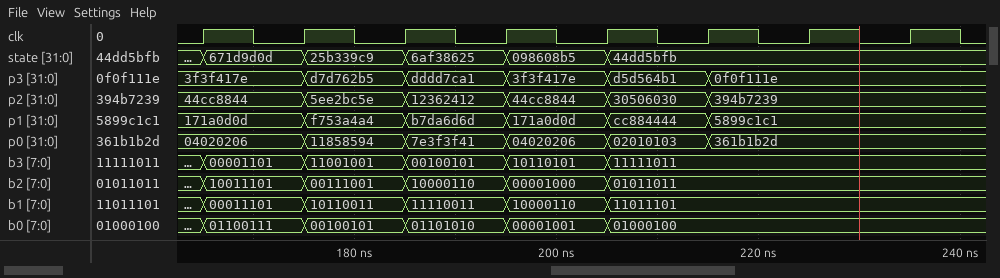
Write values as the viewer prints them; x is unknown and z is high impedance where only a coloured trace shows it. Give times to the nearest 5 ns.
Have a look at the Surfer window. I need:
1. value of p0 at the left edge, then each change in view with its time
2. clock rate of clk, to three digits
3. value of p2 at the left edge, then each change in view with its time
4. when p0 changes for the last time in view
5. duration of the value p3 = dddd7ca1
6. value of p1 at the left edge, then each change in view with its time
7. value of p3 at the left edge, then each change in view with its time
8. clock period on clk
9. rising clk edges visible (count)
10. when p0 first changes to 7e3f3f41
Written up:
04020206, 11858594 at 175 ns, 7e3f3f41 at 185 ns, 04020206 at 195 ns, 02010103 at 205 ns, 361b1b2d at 215 ns
100 MHz
44cc8844, 5ee2bc5e at 175 ns, 12362412 at 185 ns, 44cc8844 at 195 ns, 30506030 at 205 ns, 394b7239 at 215 ns
215 ns
10 ns
171a0d0d, f753a4a4 at 175 ns, b7da6d6d at 185 ns, 171a0d0d at 195 ns, cc884444 at 205 ns, 5899c1c1 at 215 ns
3f3f417e, d7d762b5 at 175 ns, dddd7ca1 at 185 ns, 3f3f417e at 195 ns, d5d564b1 at 205 ns, 0f0f111e at 215 ns
10 ns
8
185 ns
